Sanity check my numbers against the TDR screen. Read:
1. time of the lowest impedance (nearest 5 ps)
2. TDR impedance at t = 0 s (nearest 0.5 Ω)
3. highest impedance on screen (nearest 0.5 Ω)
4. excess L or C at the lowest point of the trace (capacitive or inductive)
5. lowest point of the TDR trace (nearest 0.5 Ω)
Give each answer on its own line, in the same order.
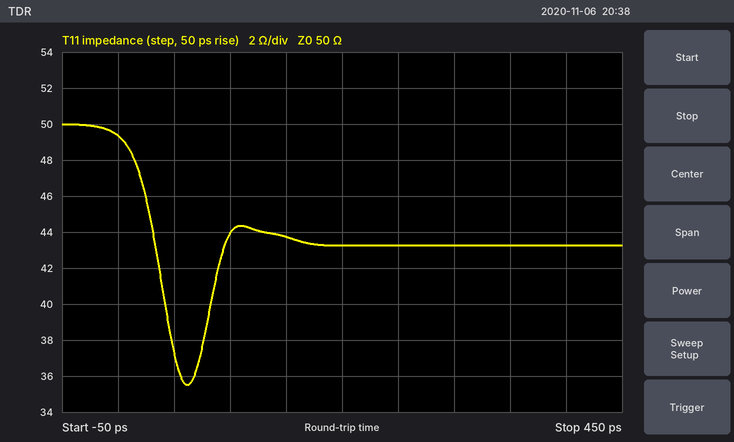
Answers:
60 ps
49.5 Ω
50.0 Ω
capacitive
35.5 Ω
